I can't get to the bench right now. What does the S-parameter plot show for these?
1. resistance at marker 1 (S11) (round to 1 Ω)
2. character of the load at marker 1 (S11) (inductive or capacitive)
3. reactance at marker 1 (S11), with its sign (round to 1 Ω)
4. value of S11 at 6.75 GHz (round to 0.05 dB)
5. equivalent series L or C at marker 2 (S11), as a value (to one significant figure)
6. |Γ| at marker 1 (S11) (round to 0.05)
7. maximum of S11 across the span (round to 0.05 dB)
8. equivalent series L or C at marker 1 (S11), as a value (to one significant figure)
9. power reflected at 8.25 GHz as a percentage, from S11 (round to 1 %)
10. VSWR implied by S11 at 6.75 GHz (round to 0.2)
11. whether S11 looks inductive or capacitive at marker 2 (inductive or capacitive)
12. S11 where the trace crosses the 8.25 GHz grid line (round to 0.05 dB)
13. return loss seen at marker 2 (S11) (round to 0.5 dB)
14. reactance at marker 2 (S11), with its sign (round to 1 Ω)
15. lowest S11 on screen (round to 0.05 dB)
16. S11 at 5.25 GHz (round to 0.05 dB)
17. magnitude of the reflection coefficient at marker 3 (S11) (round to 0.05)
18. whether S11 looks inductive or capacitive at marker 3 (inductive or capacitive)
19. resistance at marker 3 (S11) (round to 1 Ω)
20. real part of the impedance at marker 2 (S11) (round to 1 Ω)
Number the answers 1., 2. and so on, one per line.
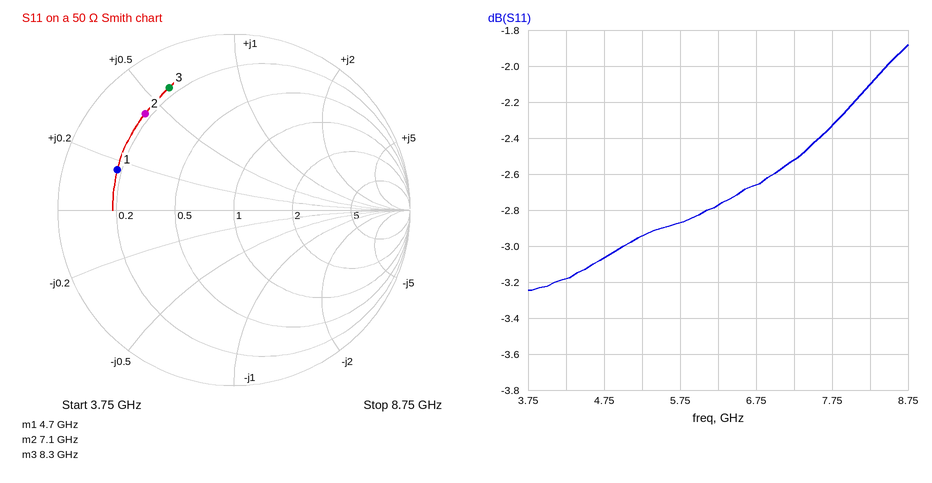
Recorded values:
1. 9 Ω
2. inductive
3. +8 Ω
4. -2.65 dB
5. 500 pH
6. 0.70
7. -1.90 dB
8. 300 pH
9. 62 %
10. 6.6
11. inductive
12. -2.10 dB
13. 2.5 dB
14. +21 Ω
15. -3.25 dB
16. -2.95 dB
17. 0.80
18. inductive
19. 8 Ω
20. 9 Ω
